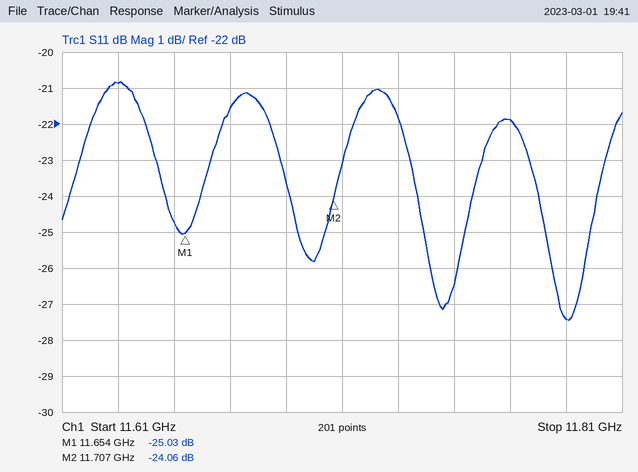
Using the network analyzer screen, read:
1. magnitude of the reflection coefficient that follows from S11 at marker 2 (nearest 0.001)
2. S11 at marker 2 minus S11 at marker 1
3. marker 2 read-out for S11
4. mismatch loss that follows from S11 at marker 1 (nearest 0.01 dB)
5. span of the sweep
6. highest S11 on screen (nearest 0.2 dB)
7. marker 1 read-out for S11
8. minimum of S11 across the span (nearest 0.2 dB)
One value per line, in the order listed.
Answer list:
0.063
0.97 dB
-24.06 dB
0.01 dB
200 MHz
-20.8 dB
-25.03 dB
-27.4 dB
